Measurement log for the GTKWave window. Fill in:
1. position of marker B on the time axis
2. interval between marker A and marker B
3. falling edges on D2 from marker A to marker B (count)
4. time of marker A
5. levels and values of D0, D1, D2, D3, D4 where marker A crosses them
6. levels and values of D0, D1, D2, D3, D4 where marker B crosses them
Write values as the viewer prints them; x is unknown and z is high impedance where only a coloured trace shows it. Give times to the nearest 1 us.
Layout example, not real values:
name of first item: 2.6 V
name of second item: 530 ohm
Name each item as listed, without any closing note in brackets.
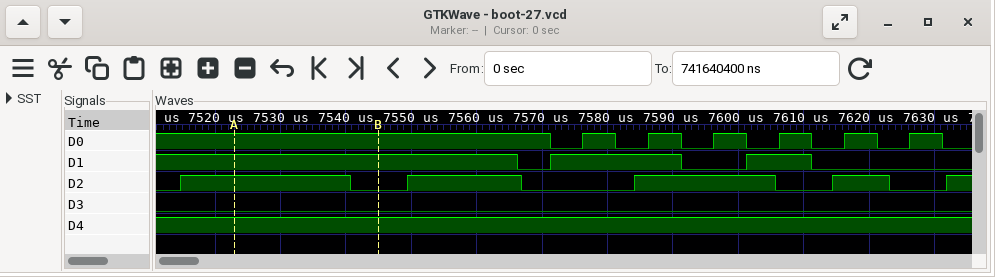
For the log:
position of marker B on the time axis: 7545 us
interval between marker A and marker B: 22 us
falling edges on D2 from marker A to marker B: 1
time of marker A: 7523 us
levels and values of D0, D1, D2, D3, D4 where marker A crosses them: D0=1, D1=1, D2=1, D3=0, D4=1
levels and values of D0, D1, D2, D3, D4 where marker B crosses them: D0=1, D1=1, D2=0, D3=0, D4=1
